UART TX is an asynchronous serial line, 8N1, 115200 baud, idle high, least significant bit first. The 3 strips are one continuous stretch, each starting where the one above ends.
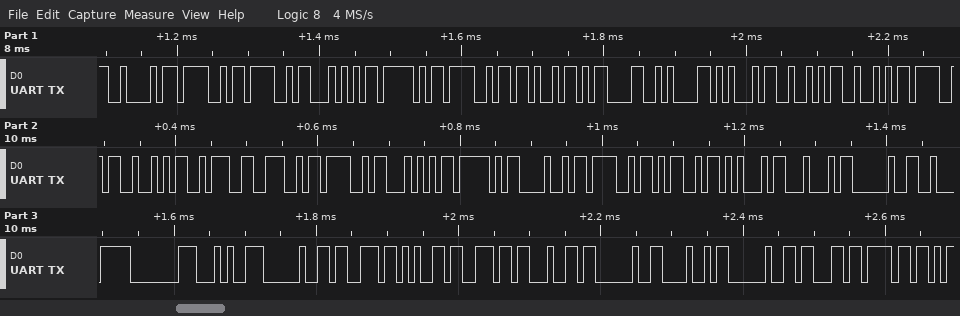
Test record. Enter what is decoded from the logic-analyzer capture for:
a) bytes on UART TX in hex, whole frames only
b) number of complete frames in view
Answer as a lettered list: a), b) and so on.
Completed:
a) 0x42 0x4F 0x4F 0x54 0x5F 0x4F 0x4B 0x0D 0x0A 0x45 0x52 0x52 0x4F 0x52 0x3A 0x4E 0x4F 0x54 0x5F 0x48 0x4F 0x4D 0x45 0x44 0x20 0xE2 0x80 0x94 0x20 0x73 0x65 0x6E 0x64 0x20 0x48 0x20 0x63 0x6F
b) 38
